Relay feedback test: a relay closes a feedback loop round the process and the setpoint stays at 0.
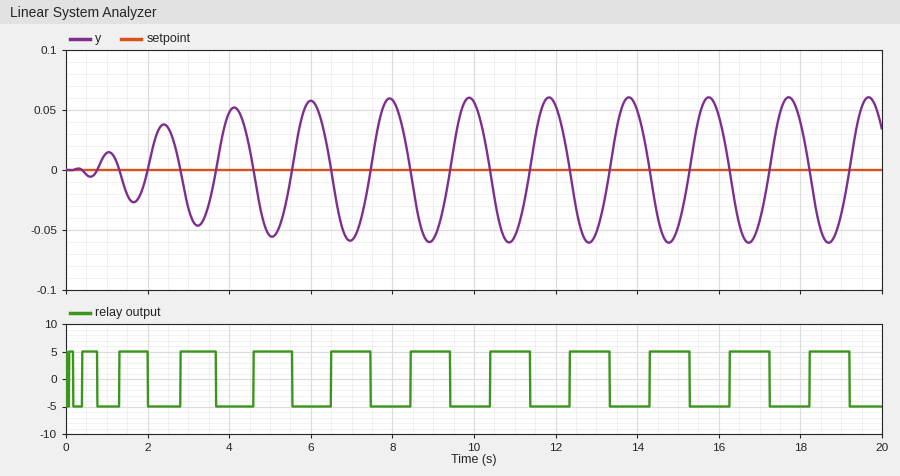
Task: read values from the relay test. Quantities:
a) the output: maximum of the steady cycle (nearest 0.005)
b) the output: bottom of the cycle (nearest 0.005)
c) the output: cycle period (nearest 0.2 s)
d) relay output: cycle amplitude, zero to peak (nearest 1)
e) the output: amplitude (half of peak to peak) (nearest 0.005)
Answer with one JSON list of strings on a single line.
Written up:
["0.060", "-0.060", "2.0 s", "5", "0.060"]
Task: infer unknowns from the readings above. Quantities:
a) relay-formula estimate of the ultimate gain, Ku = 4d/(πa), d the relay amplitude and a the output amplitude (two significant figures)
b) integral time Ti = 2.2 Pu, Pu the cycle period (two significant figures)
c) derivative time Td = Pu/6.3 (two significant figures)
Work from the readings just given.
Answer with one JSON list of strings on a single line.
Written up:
["110", "4.4 s", "0.32 s"]
